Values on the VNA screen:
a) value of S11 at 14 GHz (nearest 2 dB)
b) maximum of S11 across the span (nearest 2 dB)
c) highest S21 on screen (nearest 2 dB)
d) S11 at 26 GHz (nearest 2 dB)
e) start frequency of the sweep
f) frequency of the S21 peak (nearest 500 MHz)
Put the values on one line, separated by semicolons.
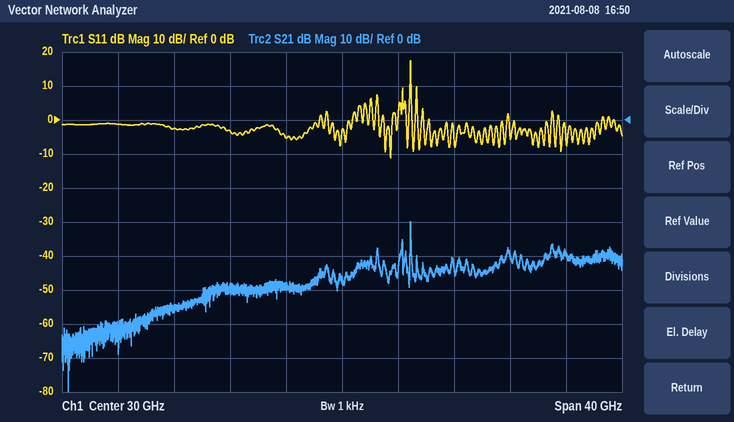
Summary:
-2 dB; 18 dB; -30 dB; -6 dB; 10 GHz; 35.0 GHz
